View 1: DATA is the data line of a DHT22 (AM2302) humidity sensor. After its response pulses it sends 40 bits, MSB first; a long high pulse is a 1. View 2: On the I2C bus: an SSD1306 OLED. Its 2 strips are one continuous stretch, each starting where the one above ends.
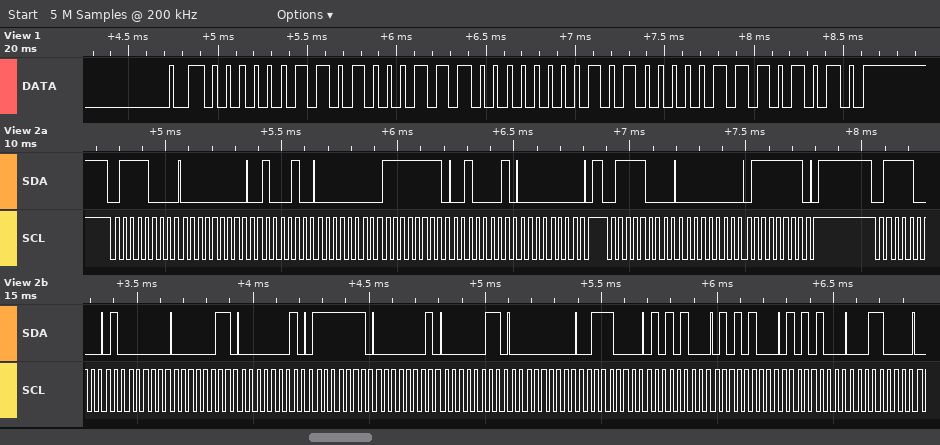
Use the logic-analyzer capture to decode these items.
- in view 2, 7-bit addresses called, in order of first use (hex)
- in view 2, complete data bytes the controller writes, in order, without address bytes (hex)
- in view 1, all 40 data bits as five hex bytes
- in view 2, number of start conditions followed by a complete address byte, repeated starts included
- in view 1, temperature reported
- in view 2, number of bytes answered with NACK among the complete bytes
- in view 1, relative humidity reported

0x3C
00 22 00 FF 21 00 00 7F 40 03 01 7F 01 03 00 38 54 54 54 18
03 47 00 A0 EA
3
16.0 °C
0
83.9 %
